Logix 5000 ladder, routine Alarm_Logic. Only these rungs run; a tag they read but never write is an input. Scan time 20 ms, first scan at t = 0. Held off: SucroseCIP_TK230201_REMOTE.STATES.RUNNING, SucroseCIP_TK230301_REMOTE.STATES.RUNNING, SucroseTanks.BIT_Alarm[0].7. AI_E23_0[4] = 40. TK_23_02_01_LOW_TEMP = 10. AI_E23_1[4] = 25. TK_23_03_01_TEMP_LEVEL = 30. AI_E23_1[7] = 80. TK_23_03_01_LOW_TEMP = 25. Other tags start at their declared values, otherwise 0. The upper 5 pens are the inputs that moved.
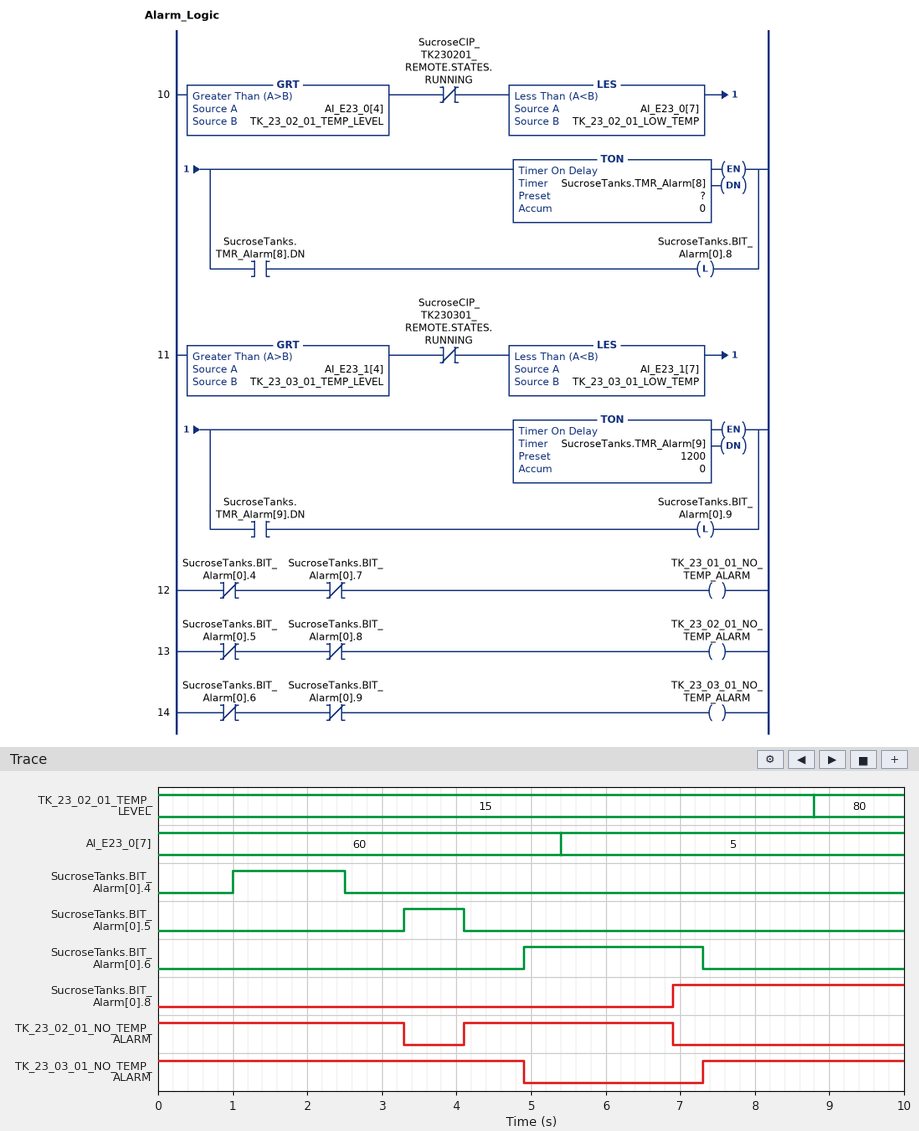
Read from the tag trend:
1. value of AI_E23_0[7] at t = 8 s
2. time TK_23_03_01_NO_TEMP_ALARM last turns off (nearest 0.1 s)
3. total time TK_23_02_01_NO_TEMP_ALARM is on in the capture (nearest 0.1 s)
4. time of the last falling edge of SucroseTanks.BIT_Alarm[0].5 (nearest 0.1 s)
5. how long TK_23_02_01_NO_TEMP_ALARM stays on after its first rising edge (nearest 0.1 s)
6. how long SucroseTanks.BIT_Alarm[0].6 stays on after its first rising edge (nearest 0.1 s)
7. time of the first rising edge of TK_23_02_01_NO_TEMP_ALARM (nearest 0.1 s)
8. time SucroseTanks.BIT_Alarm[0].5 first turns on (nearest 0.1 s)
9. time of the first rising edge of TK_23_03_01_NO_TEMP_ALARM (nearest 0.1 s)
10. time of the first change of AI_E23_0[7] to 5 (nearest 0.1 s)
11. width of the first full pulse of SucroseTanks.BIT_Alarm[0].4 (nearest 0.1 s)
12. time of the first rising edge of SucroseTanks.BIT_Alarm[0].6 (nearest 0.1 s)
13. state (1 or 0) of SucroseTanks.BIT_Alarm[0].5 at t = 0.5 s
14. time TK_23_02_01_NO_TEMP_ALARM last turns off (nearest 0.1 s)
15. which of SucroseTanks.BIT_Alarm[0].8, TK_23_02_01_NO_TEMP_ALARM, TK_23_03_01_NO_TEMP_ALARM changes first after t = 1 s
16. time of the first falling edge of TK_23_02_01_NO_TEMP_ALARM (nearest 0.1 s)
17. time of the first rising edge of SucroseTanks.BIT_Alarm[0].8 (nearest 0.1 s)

5
4.9 s
6.1 s
4.1 s
2.8 s
2.4 s
4.1 s
3.3 s
7.3 s
5.4 s
1.5 s
4.9 s
0
6.9 s
TK_23_02_01_NO_TEMP_ALARM
3.3 s
6.9 s
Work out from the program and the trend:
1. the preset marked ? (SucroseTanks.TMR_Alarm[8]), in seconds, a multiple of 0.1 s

1.5 s
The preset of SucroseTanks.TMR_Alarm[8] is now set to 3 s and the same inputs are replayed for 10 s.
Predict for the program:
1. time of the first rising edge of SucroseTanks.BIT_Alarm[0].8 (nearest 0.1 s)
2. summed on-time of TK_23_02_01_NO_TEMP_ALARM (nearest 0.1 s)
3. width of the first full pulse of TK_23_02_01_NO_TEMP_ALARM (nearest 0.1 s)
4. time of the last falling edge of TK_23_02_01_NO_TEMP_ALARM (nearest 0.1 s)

8.4 s
7.6 s
4.3 s
8.4 s
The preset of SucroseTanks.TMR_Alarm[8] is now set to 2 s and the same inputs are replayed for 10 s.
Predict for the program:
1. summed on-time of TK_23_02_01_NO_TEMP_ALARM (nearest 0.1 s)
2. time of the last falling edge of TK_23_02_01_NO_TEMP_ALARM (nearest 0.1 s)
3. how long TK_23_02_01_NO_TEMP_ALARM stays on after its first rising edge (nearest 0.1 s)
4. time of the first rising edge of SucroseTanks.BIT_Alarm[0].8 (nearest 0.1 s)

6.6 s
7.4 s
3.3 s
7.4 s
